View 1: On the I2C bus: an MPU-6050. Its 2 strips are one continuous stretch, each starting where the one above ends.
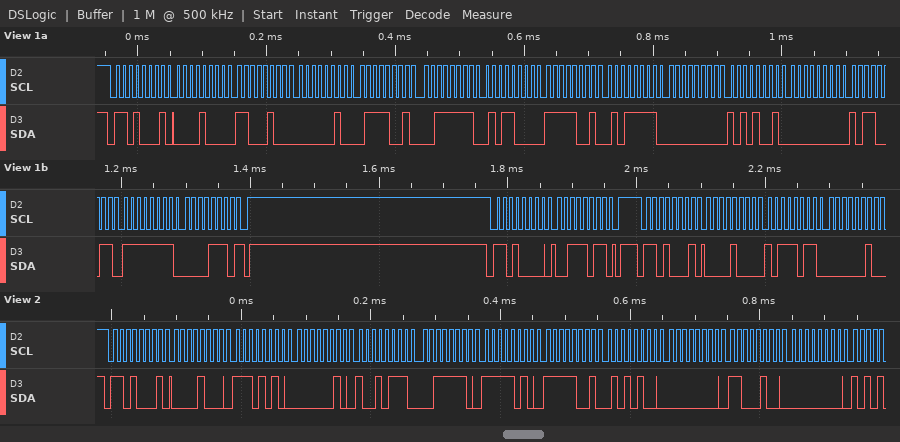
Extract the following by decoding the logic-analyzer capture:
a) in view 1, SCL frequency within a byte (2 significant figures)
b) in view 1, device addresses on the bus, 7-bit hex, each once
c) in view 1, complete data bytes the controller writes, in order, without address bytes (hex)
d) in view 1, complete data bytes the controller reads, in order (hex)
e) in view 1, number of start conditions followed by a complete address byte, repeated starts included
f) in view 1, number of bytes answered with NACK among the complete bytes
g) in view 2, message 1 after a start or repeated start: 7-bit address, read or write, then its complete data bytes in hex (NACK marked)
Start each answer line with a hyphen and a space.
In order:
- 100 kHz
- 0x68
- 3B
- 08 C4 02 79 3F 58 F9 5F 00 A9 00 B3 FF 0E 08 BB 02
- 3
- 1
- 0x68 read: 08 EA 02 97 3E FA F9 54 00 C4 00
